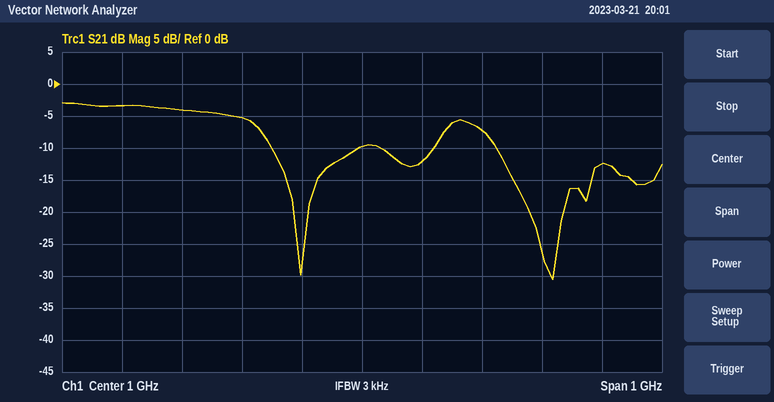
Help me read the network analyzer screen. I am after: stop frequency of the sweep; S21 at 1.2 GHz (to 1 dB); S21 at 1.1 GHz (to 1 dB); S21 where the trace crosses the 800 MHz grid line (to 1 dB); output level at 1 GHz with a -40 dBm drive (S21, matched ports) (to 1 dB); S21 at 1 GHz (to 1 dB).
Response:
1.5 GHz
-7 dB
-12 dB
-5 dB
-50 dBm
-10 dB
